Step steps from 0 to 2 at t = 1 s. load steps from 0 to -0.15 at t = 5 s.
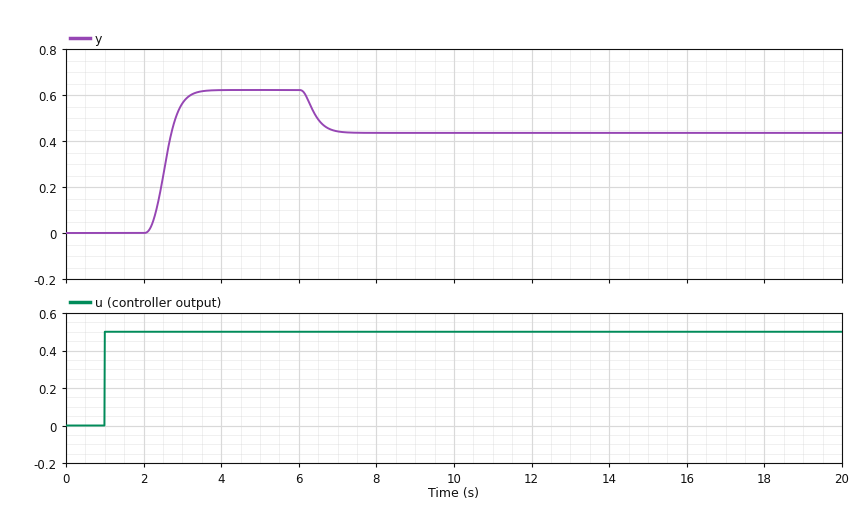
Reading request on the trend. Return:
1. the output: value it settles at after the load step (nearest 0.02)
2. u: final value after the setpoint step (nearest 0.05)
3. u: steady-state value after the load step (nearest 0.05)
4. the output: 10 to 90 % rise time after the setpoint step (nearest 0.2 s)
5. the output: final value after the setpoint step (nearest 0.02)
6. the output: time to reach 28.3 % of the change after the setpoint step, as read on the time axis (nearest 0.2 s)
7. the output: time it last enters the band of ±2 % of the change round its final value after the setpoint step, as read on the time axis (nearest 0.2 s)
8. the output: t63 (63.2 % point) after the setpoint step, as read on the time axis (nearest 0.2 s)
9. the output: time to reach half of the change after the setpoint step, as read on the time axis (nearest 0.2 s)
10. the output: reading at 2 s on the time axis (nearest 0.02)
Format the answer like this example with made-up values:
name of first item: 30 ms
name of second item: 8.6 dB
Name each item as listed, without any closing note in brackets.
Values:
the output: value it settles at after the load step: 0.44
u: final value after the setpoint step: 0.50
u: steady-state value after the load step: 0.50
the output: 10 to 90 % rise time after the setpoint step: 0.8 s
the output: final value after the setpoint step: 0.62
the output: time to reach 28.3 % of the change after the setpoint step, as read on the time axis: 2.4 s
the output: time it last enters the band of ±2 % of the change round its final value after the setpoint step, as read on the time axis: 3.4 s
the output: t63 (63.2 % point) after the setpoint step, as read on the time axis: 2.6 s
the output: time to reach half of the change after the setpoint step, as read on the time axis: 2.6 s
the output: reading at 2 s on the time axis: 0.00
